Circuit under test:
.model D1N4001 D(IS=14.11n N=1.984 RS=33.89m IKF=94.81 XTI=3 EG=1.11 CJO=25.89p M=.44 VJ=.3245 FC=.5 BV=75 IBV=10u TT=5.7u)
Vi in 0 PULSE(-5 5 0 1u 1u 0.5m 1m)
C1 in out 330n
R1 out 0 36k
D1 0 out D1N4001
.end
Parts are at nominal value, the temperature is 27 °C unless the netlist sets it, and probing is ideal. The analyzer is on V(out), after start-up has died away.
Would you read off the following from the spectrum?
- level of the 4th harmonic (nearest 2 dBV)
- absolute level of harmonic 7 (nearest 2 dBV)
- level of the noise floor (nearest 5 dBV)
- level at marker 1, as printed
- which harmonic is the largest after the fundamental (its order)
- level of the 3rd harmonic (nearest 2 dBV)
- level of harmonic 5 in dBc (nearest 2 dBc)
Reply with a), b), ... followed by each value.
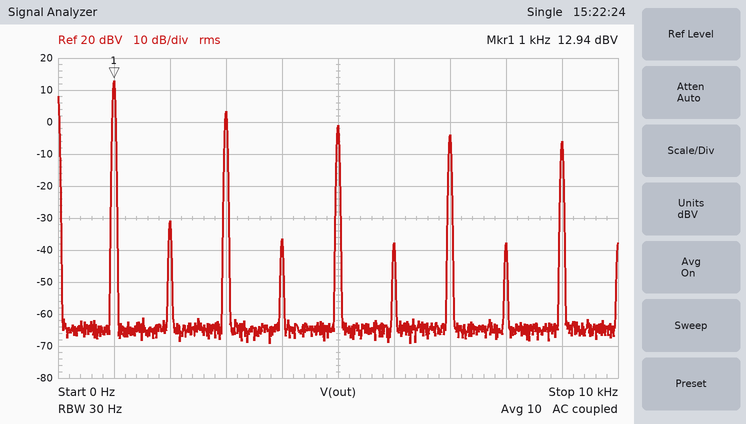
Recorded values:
a) -36 dBV
b) -4 dBV
c) -65 dBV
d) 12.94 dBV
e) 3
f) 4 dBV
g) -14 dBc
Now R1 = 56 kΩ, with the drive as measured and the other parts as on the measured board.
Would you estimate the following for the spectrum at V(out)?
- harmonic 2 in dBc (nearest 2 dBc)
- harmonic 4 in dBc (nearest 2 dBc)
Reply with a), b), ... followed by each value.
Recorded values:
a) -50 dBc
b) -52 dBc
